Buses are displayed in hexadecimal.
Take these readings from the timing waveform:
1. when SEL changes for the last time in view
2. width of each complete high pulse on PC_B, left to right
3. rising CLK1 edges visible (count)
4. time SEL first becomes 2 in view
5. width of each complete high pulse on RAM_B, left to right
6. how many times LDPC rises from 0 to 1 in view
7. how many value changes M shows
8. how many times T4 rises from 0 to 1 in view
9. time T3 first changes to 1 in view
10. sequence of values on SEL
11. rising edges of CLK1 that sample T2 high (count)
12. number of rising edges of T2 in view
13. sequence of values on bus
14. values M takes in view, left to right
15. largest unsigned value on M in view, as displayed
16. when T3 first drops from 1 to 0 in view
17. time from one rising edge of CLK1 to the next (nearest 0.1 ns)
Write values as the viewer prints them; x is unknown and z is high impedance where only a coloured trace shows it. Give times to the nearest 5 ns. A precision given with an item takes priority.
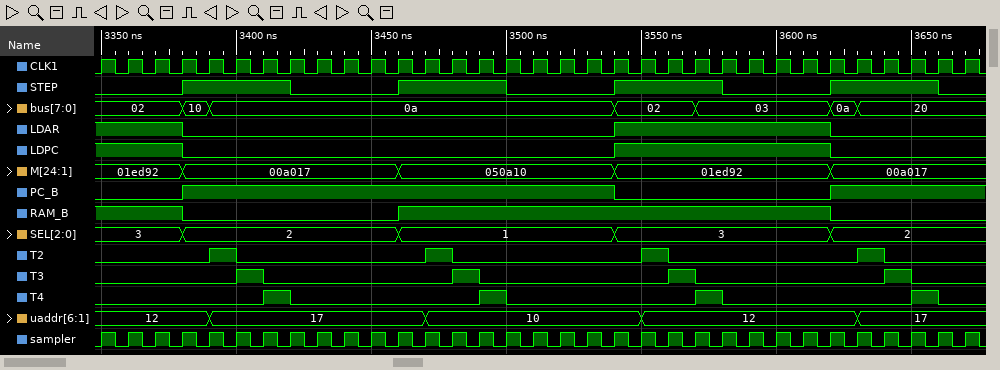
3620 ns
160 ns
33
3380 ns
160 ns
1
4
4
3400 ns
3, 2, 1, 3, 2
4
4
02, 10, 0a, 02, 03, 0a, 20
01ed92, 00a017, 050a10, 01ed92, 00a017
050a10
3410 ns
10 ns
